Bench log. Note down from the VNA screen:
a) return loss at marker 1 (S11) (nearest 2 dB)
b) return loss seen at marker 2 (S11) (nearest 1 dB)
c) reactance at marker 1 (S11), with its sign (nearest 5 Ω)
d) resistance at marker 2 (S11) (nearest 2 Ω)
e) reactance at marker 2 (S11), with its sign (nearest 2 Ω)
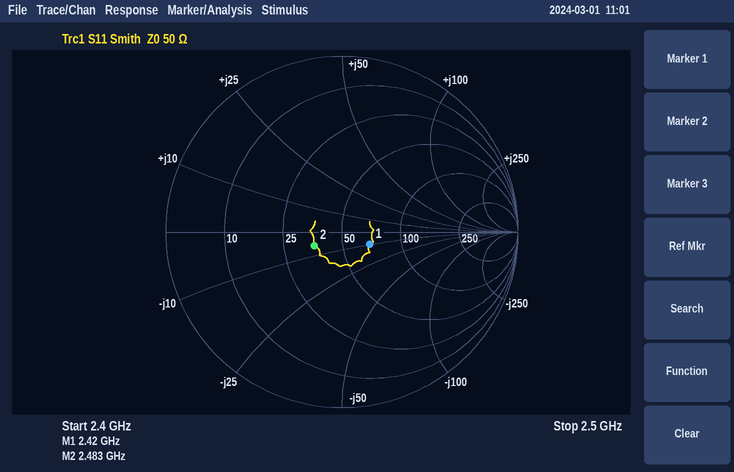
16 dB
15 dB
-10 Ω
36 Ω
-6 Ω
